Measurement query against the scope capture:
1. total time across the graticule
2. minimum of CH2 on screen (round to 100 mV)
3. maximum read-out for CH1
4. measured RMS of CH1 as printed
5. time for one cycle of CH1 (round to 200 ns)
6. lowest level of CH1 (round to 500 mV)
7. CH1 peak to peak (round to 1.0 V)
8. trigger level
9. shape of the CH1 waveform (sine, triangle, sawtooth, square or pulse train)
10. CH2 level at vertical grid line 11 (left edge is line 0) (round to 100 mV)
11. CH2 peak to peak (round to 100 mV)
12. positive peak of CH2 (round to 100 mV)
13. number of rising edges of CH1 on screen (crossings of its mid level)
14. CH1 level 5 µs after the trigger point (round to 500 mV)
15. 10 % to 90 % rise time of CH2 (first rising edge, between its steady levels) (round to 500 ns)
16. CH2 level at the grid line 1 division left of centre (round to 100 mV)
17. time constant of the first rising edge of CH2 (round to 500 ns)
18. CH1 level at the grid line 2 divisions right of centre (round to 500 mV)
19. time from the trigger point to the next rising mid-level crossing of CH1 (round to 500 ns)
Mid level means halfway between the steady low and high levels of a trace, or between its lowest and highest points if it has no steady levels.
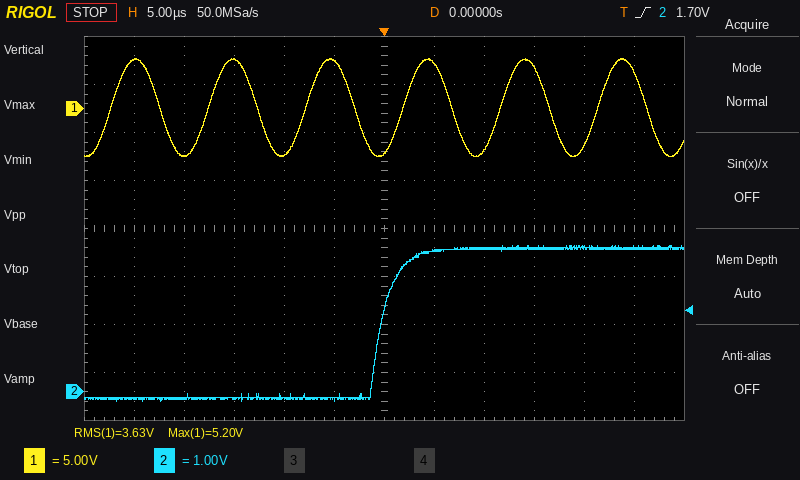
60 µs
-200 mV
5.20 V
3.63 V
9.8 µs
-5.0 V
10.0 V
1.70 V
sine
3.0 V
3.2 V
3.0 V
6
4.5 V
3.5 µs
-200 mV
1.5 µs
-4.5 V
2.0 µs
